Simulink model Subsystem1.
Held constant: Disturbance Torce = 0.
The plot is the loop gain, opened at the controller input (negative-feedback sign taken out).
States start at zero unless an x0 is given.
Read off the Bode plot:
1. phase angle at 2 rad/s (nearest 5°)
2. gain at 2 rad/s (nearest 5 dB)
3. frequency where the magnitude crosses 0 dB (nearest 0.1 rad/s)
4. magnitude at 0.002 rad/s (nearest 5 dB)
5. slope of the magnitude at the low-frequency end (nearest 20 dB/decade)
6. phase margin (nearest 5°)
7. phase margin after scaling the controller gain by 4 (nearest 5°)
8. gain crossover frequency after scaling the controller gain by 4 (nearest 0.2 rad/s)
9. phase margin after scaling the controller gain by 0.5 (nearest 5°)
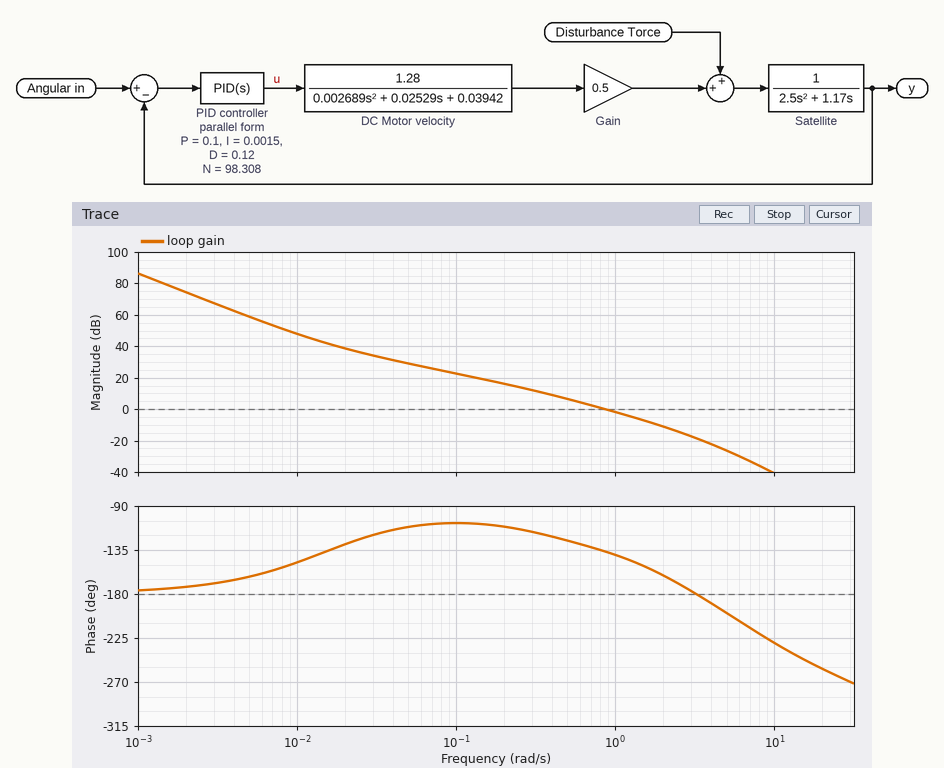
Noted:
-160°
-10 dB
0.9 rad/s
75 dB
-40 dB/decade
45°
15°
2.2 rad/s
55°
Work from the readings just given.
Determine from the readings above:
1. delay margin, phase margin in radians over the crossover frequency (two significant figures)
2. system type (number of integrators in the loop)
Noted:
0.87 s
2
